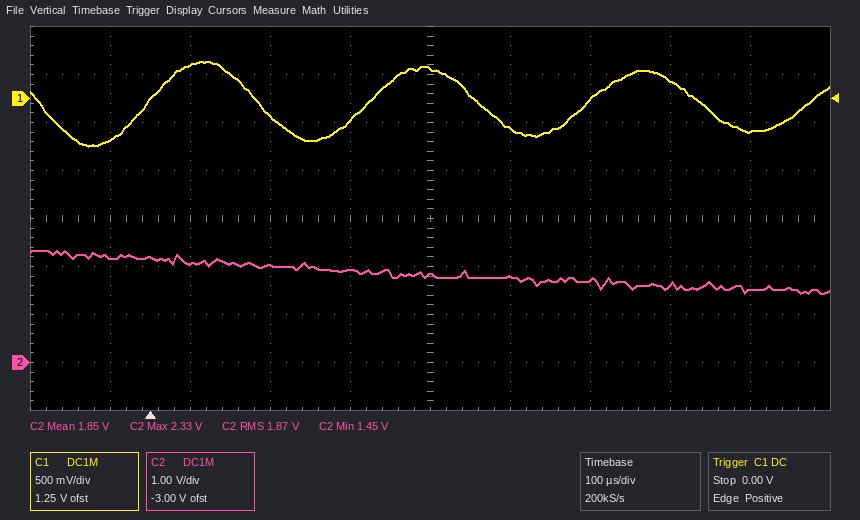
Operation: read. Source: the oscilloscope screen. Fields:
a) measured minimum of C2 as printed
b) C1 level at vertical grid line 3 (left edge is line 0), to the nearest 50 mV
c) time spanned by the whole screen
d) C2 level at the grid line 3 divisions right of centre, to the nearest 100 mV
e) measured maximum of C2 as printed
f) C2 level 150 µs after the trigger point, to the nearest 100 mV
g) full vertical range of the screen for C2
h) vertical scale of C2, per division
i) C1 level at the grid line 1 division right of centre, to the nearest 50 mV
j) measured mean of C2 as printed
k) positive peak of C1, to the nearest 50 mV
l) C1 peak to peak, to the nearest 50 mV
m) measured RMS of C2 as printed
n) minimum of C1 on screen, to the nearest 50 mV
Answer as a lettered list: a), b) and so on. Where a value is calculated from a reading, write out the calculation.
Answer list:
a) 1.45 V
b) -200 mV
c) 1 ms
d) 1.6 V
e) 2.33 V
f) 2.0 V
g) 8 V
h) 1 V
i) -300 mV
j) 1.85 V
k) 400 mV
l) 400 mV − (-500 mV) = 900 mV
m) 1.87 V
n) -500 mV
